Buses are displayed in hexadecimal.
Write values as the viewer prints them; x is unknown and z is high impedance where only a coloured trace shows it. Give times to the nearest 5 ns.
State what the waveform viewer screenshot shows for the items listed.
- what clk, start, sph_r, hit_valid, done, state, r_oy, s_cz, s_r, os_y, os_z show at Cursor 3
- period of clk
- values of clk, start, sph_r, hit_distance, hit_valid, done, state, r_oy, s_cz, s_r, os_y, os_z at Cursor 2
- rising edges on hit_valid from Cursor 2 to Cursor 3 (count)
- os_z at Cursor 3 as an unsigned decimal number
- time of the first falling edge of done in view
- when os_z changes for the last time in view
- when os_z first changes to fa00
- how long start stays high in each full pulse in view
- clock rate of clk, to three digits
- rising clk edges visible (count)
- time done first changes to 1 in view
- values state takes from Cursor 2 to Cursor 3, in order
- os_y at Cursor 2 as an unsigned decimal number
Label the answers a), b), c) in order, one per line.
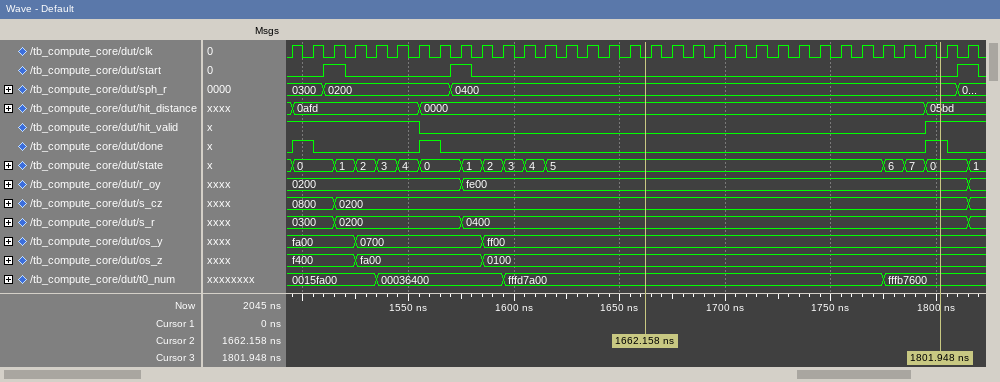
a) clk=0, start=0, sph_r=0400, hit_valid=1, done=1, state=0, r_oy=fe00, s_cz=0200, s_r=0400, os_y=ff00, os_z=0100
b) 10 ns
c) clk=0, start=0, sph_r=0400, hit_distance=0000, hit_valid=0, done=0, state=5, r_oy=fe00, s_cz=0200, s_r=0400, os_y=ff00, os_z=0100
d) 1
e) 256
f) 1505 ns
g) 1585 ns
h) 1525 ns
i) 10 ns, 10 ns, 10 ns
j) 100 MHz
k) 33
l) 1495 ns
m) 5, 6, 7, 0
n) 65280
